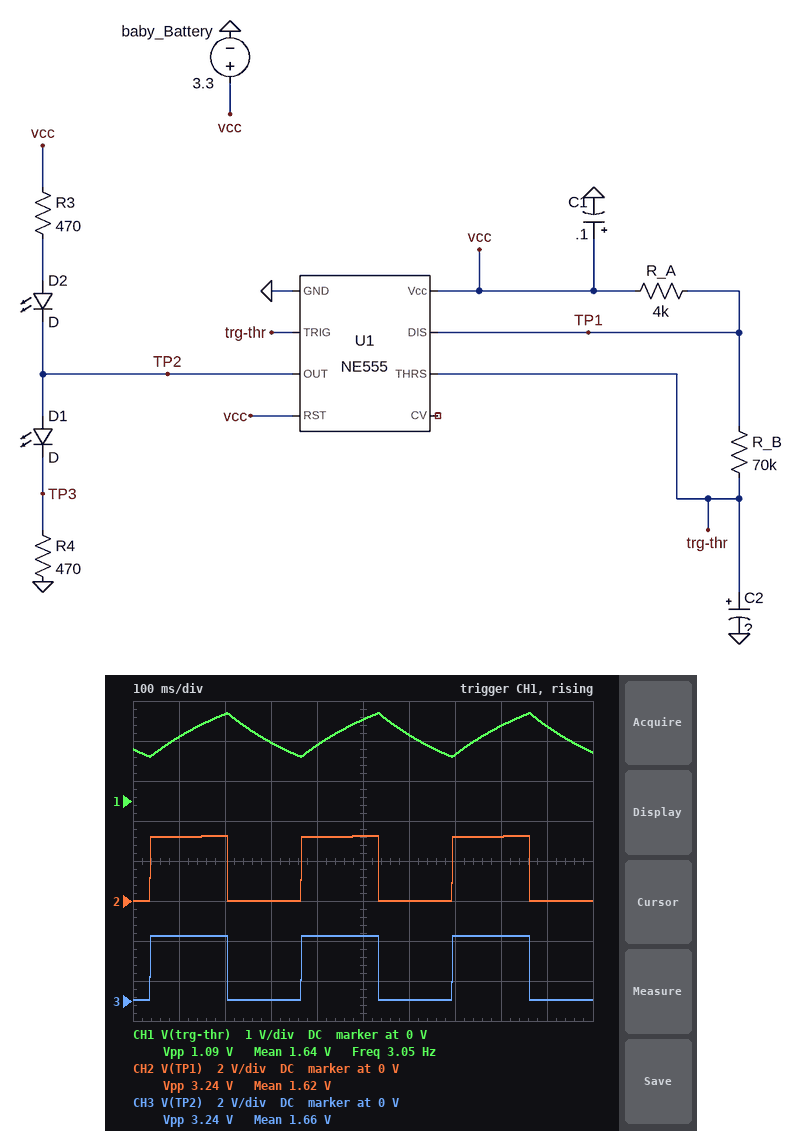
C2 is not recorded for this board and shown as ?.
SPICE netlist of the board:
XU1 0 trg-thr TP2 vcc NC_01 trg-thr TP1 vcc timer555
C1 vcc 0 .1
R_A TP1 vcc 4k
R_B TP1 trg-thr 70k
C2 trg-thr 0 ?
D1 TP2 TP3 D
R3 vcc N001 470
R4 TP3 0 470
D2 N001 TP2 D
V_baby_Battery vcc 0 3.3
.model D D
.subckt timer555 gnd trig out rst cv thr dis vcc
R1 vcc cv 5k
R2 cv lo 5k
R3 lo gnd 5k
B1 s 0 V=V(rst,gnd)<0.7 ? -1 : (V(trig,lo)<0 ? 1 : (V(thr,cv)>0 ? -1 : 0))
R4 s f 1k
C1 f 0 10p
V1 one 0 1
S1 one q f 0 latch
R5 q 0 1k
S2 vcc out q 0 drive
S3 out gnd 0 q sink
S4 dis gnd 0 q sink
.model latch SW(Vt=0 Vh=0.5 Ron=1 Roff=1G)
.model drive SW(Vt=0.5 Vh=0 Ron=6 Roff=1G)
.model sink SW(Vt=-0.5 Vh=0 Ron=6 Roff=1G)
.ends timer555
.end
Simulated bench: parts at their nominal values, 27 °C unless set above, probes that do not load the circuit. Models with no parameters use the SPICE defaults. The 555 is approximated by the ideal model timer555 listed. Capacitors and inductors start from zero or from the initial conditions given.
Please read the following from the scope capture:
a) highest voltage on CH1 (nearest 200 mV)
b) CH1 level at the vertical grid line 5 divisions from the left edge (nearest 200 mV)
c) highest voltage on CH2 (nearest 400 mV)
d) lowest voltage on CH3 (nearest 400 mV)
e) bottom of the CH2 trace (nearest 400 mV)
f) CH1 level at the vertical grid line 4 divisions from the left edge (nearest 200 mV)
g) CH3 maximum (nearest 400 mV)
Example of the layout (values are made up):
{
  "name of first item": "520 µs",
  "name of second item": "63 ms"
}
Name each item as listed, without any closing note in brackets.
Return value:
{
  "highest voltage on CH1": "2.2 V",
  "CH1 level at the vertical grid line 5 divisions from the left edge": "2.0 V",
  "highest voltage on CH2": "3.2 V",
  "lowest voltage on CH3": "0 V",
  "bottom of the CH2 trace": "0 V",
  "CH1 level at the vertical grid line 4 divisions from the left edge": "1.4 V",
  "CH3 maximum": "3.2 V"
}
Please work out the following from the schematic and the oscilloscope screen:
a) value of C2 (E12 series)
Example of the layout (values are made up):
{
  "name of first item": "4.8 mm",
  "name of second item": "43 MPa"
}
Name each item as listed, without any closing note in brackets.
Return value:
{
  "value of C2": "3.3 µF"
}
